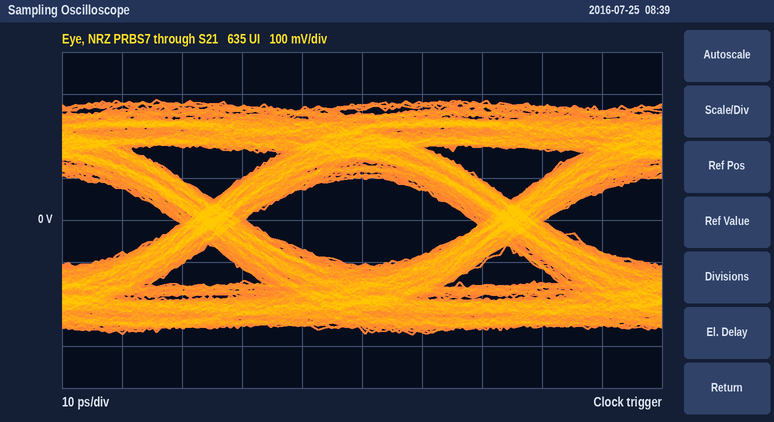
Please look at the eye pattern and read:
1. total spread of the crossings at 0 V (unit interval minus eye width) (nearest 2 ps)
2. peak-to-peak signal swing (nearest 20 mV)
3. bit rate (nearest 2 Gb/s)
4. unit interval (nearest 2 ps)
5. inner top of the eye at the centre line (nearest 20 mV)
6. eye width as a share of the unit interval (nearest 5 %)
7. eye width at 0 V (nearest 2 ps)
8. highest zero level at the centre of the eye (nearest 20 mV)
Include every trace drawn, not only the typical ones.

12 ps
560 mV
20 Gb/s
50 ps
100 mV
75 %
38 ps
-100 mV
